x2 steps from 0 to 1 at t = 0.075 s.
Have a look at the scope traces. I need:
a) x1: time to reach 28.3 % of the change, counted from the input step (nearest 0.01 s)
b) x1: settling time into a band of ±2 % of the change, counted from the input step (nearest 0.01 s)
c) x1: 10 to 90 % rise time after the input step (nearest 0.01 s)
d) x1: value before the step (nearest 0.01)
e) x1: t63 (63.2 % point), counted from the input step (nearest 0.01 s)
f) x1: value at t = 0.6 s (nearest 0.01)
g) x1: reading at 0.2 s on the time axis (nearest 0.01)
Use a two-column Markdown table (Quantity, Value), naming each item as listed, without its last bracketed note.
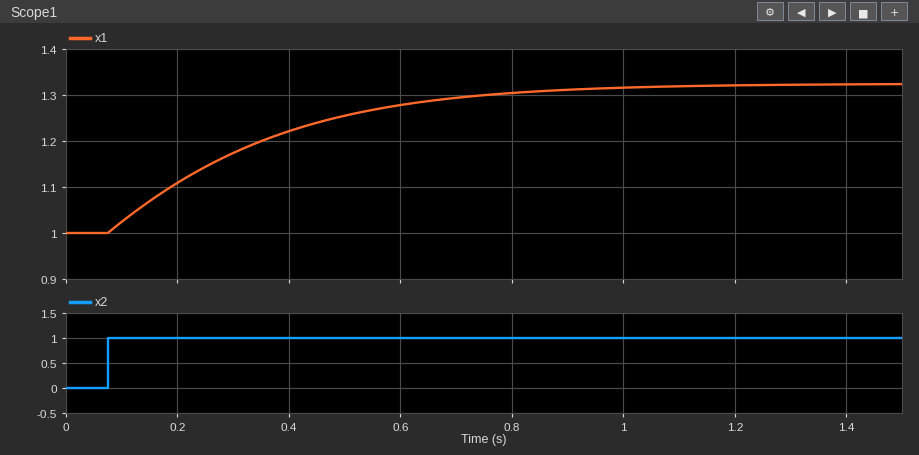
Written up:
| Quantity | Value |
|---|---|
| x1: time to reach 28.3 % of the change, counted from the input step | 0.10 s |
| x1: settling time into a band of ±2 % of the change, counted from the input step | 1.00 s |
| x1: 10 to 90 % rise time after the input step | 0.58 s |
| x1: value before the step | 1.00 |
| x1: t63 (63.2 % point), counted from the input step | 0.29 s |
| x1: value at t = 0.6 s | 1.28 |
| x1: reading at 0.2 s on the time axis | 1.11 |
